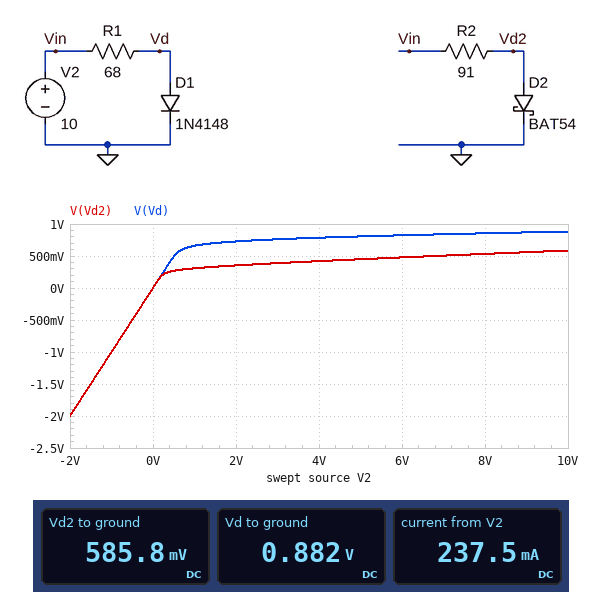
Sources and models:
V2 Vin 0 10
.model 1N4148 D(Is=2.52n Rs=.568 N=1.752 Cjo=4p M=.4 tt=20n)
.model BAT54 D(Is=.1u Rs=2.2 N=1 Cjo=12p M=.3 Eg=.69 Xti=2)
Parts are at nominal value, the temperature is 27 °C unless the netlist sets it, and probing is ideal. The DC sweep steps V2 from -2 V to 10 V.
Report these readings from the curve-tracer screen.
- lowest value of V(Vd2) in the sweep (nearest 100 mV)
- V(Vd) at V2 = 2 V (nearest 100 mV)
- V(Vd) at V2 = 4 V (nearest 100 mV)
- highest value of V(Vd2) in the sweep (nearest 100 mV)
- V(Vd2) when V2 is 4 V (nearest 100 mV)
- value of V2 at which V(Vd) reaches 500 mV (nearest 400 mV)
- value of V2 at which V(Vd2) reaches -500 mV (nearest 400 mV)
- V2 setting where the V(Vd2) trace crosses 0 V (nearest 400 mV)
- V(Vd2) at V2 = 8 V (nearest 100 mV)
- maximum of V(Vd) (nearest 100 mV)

-2.0 V
700 mV
800 mV
600 mV
400 mV
400 mV
-400 mV
0 V
500 mV
900 mV
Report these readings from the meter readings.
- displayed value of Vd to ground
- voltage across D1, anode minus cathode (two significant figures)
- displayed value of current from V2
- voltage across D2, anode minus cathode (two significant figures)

0.882 V
880 mV
237.5 mA
590 mV
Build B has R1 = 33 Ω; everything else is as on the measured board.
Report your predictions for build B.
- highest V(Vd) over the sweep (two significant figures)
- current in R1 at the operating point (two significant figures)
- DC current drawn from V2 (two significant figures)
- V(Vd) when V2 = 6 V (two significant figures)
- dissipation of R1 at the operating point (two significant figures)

990 mV
270 mA
380 mA
900 mV
2.5 W
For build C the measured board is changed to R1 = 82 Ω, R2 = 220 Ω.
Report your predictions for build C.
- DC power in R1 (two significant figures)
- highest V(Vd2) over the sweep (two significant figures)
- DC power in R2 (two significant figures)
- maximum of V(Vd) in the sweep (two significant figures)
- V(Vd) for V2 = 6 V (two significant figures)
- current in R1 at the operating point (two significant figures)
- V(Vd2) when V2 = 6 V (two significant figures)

1.0 W
430 mV
420 mW
860 mV
810 mV
110 mA
380 mV
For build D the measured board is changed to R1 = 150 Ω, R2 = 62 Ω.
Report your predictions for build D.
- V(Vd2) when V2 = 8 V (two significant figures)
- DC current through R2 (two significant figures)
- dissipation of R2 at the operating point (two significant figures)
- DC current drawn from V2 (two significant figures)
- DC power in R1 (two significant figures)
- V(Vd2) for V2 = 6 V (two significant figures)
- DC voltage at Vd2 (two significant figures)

620 mV
150 mA
1.4 W
210 mA
560 mW
550 mV
700 mV
